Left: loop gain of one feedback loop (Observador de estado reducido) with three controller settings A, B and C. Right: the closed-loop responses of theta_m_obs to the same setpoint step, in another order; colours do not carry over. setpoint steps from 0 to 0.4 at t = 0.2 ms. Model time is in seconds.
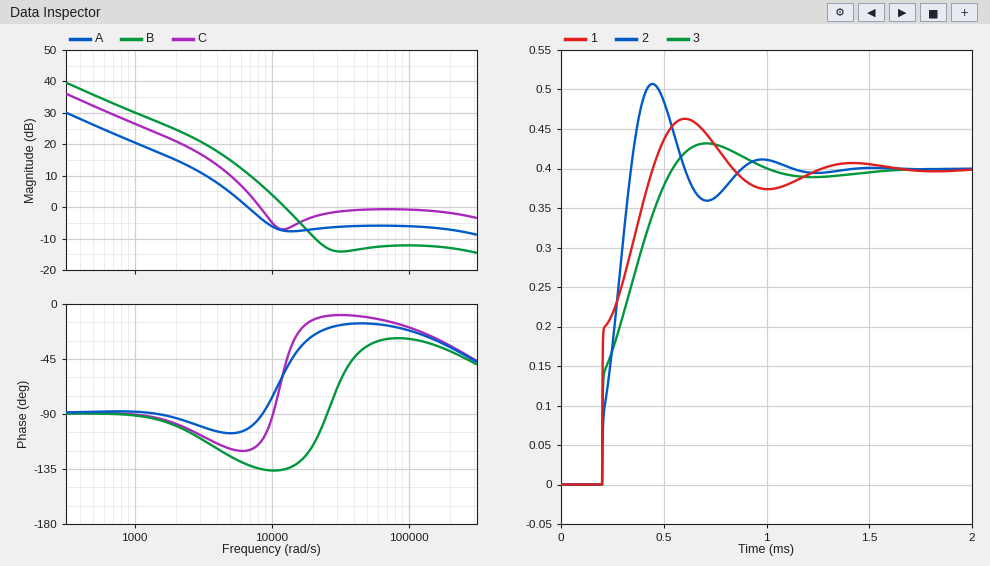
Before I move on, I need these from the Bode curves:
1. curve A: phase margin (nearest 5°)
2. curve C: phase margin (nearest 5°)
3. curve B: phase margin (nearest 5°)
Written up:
80°
65°
45°
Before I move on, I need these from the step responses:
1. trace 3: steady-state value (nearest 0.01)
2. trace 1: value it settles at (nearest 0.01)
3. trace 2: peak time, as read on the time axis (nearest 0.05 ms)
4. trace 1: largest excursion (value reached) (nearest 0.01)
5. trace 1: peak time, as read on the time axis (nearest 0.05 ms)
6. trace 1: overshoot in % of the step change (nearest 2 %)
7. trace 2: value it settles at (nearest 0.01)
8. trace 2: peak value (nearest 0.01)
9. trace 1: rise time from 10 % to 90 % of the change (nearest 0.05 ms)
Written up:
0.40
0.40
0.45 ms
0.46
0.60 ms
16 %
0.40
0.51
0.20 ms
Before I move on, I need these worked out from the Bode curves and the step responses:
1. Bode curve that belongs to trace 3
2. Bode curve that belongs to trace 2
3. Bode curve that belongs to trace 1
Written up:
A
B
C
